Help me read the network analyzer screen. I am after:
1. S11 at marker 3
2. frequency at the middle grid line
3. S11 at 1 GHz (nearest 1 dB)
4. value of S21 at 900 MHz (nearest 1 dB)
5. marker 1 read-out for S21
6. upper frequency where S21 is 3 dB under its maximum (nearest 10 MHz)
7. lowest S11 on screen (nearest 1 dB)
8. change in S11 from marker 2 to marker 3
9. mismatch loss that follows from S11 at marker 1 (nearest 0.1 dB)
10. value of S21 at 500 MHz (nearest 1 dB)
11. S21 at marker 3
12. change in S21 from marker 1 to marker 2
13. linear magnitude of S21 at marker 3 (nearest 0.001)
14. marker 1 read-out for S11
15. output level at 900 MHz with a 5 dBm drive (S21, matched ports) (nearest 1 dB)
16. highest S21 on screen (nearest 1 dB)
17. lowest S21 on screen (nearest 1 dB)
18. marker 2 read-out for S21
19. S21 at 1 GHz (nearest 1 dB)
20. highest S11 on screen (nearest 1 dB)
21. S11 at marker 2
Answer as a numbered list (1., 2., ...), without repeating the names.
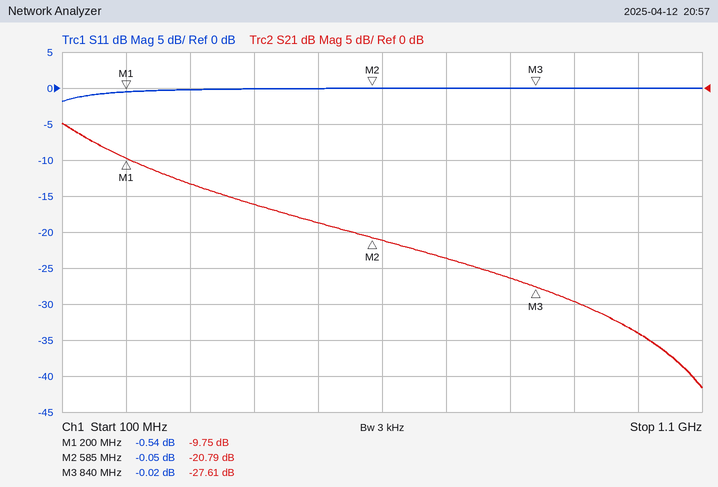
1. -0.02 dB
2. 600 MHz
3. 0 dB
4. -30 dB
5. -9.75 dB
6. 160 MHz
7. -2 dB
8. 0.03 dB
9. 9.3 dB
10. -19 dB
11. -27.61 dB
12. -11.04 dB
13. 0.042
14. -0.54 dB
15. -25 dBm
16. -5 dB
17. -42 dB
18. -20.79 dB
19. -34 dB
20. 0 dB
21. -0.05 dB
